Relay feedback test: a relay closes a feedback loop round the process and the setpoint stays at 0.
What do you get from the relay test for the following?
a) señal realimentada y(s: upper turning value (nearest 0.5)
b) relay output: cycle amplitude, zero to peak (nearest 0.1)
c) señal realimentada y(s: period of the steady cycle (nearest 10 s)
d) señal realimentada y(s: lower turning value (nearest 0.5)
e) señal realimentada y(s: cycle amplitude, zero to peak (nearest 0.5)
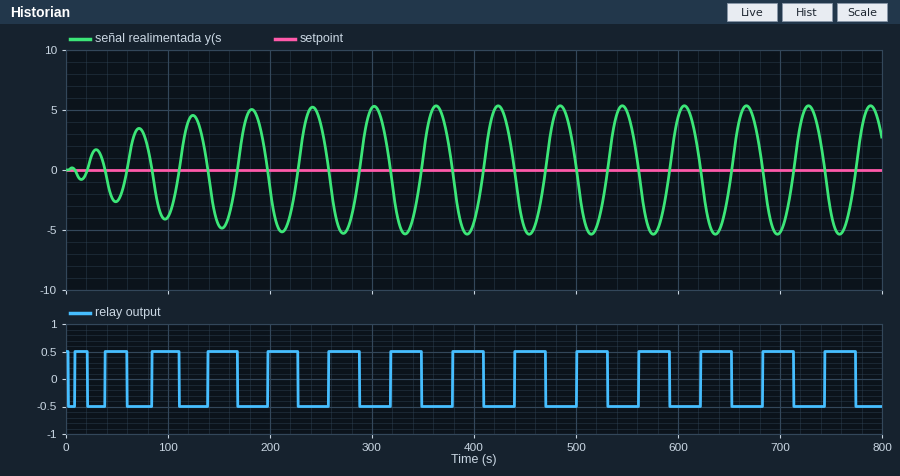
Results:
5.5
0.5
60 s
-5.5
5.5
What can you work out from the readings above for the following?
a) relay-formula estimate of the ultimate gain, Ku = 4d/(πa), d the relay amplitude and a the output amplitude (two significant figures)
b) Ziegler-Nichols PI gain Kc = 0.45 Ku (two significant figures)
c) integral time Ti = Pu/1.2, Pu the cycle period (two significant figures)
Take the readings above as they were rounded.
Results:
0.12
0.054
50 s
